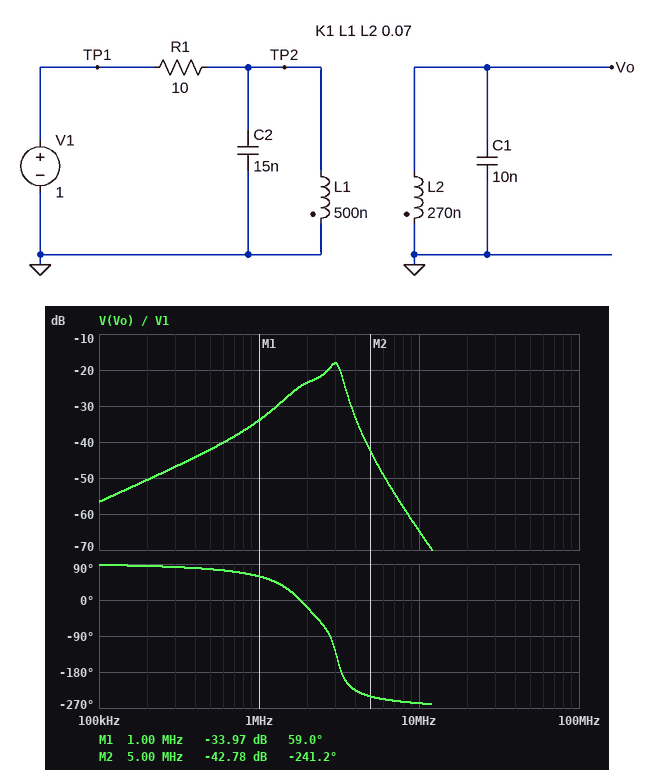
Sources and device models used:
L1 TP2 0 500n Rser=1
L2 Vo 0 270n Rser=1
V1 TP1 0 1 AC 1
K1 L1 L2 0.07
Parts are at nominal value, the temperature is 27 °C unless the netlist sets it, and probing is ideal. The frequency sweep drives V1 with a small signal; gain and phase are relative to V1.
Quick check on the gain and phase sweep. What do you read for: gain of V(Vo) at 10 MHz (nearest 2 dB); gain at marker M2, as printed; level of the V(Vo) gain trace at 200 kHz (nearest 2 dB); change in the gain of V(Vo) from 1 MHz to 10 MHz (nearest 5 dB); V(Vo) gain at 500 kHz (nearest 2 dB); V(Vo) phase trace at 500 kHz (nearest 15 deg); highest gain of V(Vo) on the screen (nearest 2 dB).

-64 dB
-42.78 dB
-50 dB
-30 dB
-42 dB
75 deg
-18 dB
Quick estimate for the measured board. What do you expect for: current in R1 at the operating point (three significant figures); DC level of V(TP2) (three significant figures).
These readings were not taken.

90.9 mA
90.9 mV
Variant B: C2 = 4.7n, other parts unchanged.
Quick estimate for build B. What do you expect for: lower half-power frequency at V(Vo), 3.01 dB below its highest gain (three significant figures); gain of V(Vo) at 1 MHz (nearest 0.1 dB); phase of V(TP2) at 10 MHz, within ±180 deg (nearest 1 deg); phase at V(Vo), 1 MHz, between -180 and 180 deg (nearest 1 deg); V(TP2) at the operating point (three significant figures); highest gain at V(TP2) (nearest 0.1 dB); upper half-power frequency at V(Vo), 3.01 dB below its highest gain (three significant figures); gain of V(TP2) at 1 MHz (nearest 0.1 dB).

2.75 MHz
-35.4 dB
-69 deg
67 deg
90.9 mV
-0.8 dB
3.34 MHz
-10.2 dB
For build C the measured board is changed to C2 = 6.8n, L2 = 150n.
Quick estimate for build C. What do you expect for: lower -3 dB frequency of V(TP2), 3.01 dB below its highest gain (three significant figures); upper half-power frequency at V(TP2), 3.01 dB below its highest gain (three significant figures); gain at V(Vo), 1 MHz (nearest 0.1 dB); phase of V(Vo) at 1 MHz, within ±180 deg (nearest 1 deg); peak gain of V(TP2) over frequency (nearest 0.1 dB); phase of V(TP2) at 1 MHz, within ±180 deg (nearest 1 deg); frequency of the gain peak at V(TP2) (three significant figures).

1.81 MHz
4.47 MHz
-38.1 dB
66 deg
-1.1 dB
52 deg
2.85 MHz
